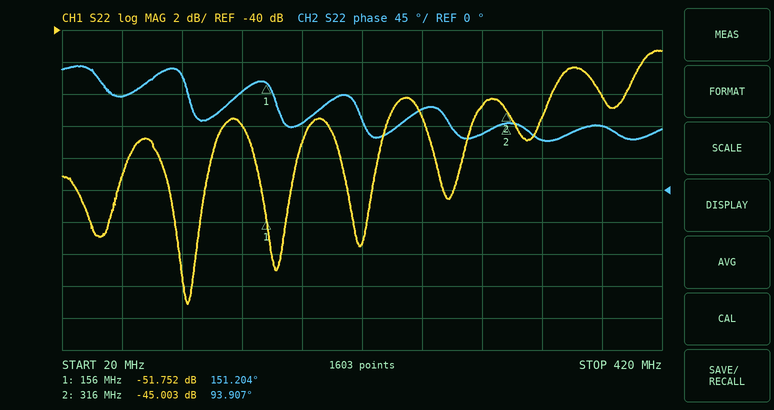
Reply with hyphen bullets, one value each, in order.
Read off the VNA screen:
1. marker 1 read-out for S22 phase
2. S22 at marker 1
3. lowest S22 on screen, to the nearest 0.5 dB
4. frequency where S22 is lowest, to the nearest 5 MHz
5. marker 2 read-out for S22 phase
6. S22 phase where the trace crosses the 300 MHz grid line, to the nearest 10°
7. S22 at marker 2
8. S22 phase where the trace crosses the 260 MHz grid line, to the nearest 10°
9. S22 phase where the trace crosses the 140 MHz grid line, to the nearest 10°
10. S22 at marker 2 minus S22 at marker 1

- 151.204°
- -51.752 dB
- -57.0 dB
- 105 MHz
- 93.907°
- 80°
- -45.003 dB
- 110°
- 140°
- 6.749 dB
